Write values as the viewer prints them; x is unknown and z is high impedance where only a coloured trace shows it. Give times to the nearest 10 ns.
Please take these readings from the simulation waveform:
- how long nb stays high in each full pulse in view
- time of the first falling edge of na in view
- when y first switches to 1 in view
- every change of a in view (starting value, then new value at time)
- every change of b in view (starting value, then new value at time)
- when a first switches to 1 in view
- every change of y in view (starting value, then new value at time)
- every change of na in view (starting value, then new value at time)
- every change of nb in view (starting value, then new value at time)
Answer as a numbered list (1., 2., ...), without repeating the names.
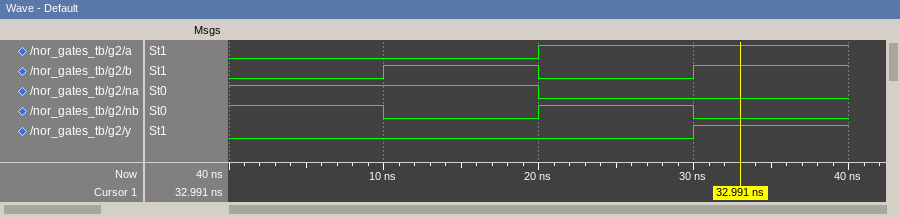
1. 10 ns
2. 20 ns
3. 30 ns
4. 0, 1 at 20 ns
5. 0, 1 at 10 ns, 0 at 20 ns, 1 at 30 ns
6. 20 ns
7. 0, 1 at 30 ns
8. 1, 0 at 20 ns
9. 1, 0 at 10 ns, 1 at 20 ns, 0 at 30 ns
